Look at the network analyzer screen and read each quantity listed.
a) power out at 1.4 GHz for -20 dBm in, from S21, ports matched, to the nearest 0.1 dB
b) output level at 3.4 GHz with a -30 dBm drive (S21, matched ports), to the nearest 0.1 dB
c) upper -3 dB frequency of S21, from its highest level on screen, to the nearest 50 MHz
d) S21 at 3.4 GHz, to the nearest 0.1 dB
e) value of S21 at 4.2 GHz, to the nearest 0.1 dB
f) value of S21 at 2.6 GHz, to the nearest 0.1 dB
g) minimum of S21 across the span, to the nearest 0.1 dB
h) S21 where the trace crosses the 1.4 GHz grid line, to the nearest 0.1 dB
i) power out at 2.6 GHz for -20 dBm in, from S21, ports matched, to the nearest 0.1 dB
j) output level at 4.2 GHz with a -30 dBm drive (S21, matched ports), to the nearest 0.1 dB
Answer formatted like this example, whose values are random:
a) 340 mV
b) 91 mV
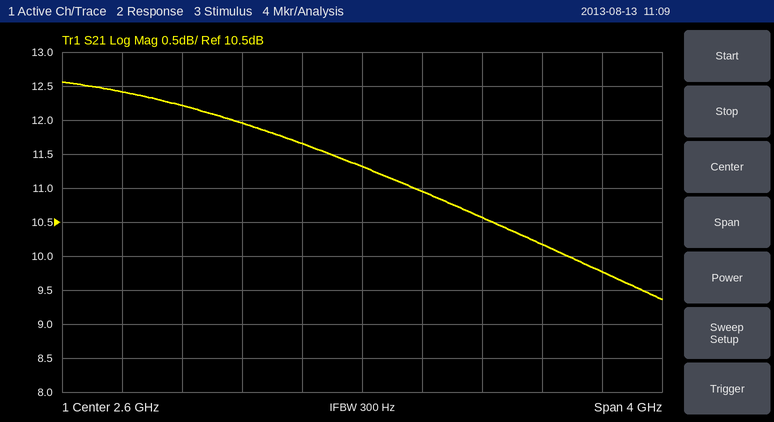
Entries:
a) -7.8 dBm
b) -19.4 dBm
c) 4.40 GHz
d) 10.6 dB
e) 9.8 dB
f) 11.3 dB
g) 9.4 dB
h) 12.2 dB
i) -8.7 dBm
j) -20.2 dBm
